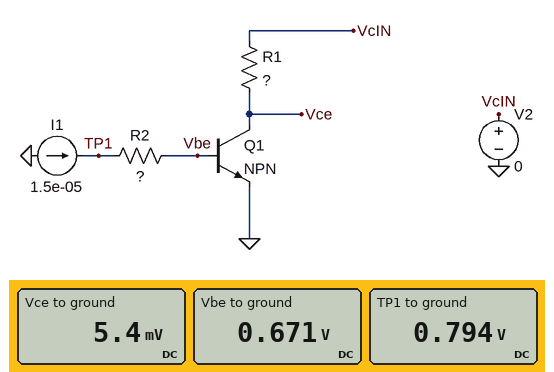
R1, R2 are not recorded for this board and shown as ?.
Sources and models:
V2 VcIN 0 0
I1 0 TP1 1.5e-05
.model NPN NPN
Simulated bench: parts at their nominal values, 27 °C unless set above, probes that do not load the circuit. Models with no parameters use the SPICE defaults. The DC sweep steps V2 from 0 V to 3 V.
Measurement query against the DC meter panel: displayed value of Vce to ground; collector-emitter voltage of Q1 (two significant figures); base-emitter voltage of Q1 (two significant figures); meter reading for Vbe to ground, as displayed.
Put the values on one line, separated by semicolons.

5.4 mV; 5.4 mV; 670 mV; 0.671 V
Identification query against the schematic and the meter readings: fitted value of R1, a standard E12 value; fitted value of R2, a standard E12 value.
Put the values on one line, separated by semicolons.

470 Ω; 8.2 kΩ
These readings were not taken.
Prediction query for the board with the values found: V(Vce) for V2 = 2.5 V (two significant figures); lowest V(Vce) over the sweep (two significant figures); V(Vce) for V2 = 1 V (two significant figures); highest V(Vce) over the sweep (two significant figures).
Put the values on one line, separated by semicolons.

1.8 V; 5.4 mV; 300 mV; 2.3 V
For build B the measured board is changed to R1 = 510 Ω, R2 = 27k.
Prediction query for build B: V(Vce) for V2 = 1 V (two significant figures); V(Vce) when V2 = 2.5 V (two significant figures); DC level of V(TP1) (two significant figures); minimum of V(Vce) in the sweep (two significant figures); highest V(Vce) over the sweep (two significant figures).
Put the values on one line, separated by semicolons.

240 mV; 1.7 V; 1.1 V; 5.7 mV; 2.2 V
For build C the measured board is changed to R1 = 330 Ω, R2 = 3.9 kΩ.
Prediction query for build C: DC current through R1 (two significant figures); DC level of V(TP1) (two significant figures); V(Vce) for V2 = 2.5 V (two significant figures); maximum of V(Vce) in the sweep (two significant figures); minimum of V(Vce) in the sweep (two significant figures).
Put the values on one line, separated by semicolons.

12 µA; 730 mV; 2.0 V; 2.5 V; 4.1 mV
